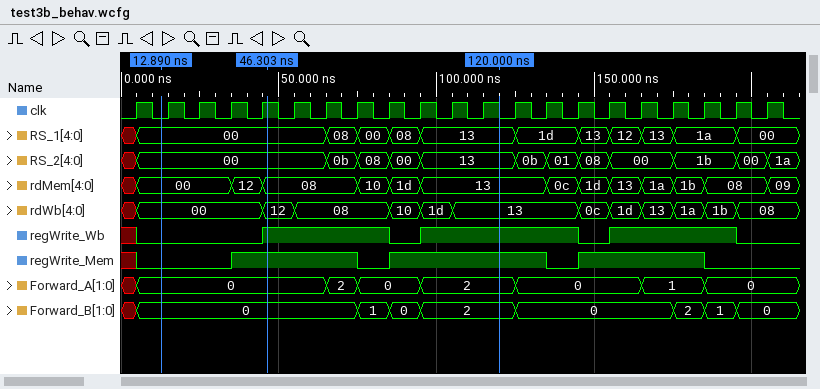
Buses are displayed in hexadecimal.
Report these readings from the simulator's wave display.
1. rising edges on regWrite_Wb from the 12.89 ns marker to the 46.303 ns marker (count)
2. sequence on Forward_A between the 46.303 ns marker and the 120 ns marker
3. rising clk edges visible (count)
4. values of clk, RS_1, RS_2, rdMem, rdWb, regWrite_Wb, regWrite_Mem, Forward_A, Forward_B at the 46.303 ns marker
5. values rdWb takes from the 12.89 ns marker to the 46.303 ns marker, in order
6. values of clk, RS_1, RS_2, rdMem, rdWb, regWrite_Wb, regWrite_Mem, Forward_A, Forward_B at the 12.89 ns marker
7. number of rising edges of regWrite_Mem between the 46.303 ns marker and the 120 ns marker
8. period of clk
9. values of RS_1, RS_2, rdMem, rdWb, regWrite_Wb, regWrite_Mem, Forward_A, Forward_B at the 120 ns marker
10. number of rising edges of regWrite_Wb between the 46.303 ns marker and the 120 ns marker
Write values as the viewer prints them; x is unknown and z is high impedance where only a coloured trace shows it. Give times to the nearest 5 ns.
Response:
1
0, 2, 0, 2
21
clk=1, RS_1=00, RS_2=00, rdMem=08, rdWb=12, regWrite_Wb=1, regWrite_Mem=1, Forward_A=0, Forward_B=0
00, 12
clk=0, RS_1=00, RS_2=00, rdMem=00, rdWb=00, regWrite_Wb=0, regWrite_Mem=0, Forward_A=0, Forward_B=0
1
10 ns
RS_1=13, RS_2=13, rdMem=13, rdWb=13, regWrite_Wb=1, regWrite_Mem=1, Forward_A=2, Forward_B=2
1
